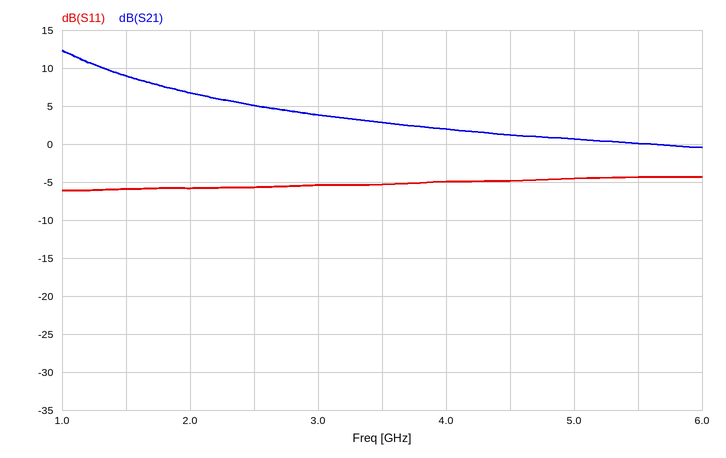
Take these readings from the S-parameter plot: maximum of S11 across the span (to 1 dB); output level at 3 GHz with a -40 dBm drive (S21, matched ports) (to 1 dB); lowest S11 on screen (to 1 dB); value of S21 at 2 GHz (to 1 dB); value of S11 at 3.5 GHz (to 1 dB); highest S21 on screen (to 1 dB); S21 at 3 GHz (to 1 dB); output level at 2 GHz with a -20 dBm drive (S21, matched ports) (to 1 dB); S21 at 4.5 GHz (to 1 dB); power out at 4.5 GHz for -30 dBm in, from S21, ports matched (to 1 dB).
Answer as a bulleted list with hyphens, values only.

- -4 dB
- -36 dBm
- -6 dB
- 7 dB
- -5 dB
- 12 dB
- 4 dB
- -13 dBm
- 1 dB
- -29 dBm
